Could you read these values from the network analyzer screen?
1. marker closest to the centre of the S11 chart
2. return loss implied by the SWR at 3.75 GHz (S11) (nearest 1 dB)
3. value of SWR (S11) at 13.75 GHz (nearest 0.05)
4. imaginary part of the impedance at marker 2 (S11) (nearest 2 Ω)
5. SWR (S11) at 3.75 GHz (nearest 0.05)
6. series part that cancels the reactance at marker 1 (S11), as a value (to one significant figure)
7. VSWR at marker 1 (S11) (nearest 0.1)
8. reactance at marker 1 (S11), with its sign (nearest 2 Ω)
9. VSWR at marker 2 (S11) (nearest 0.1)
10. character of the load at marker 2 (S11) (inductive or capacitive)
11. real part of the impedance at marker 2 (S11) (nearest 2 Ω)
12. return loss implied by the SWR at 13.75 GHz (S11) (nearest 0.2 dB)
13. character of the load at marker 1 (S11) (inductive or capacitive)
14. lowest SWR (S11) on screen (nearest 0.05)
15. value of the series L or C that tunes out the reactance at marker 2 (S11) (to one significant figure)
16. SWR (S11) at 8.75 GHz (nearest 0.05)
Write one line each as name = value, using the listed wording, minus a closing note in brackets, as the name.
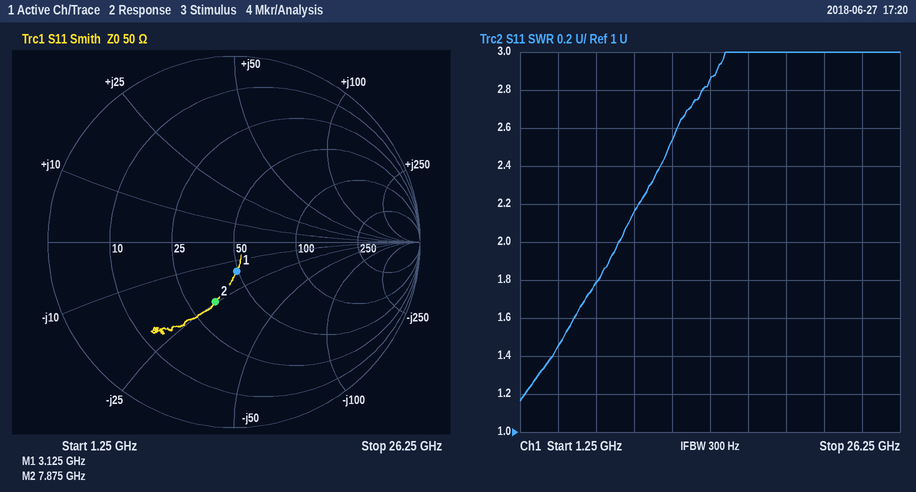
marker closest to the centre of the S11 chart = marker 1
return loss implied by the SWR at 3.75 GHz (S11) = 15 dB
value of SWR (S11) at 13.75 GHz = 2.85
imaginary part of the impedance at marker 2 (S11) = -24 Ω
SWR (S11) at 3.75 GHz = 1.45
series part that cancels the reactance at marker 1 (S11), as a value = 800 pH
VSWR at marker 1 (S11) = 1.4
reactance at marker 1 (S11), with its sign = -16 Ω
VSWR at marker 2 (S11) = 2.0
character of the load at marker 2 (S11) = capacitive
real part of the impedance at marker 2 (S11) = 34 Ω
return loss implied by the SWR at 13.75 GHz (S11) = 6.4 dB
character of the load at marker 1 (S11) = capacitive
lowest SWR (S11) on screen = 1.15
value of the series L or C that tunes out the reactance at marker 2 (S11) = 500 pH
SWR (S11) at 8.75 GHz = 2.15
